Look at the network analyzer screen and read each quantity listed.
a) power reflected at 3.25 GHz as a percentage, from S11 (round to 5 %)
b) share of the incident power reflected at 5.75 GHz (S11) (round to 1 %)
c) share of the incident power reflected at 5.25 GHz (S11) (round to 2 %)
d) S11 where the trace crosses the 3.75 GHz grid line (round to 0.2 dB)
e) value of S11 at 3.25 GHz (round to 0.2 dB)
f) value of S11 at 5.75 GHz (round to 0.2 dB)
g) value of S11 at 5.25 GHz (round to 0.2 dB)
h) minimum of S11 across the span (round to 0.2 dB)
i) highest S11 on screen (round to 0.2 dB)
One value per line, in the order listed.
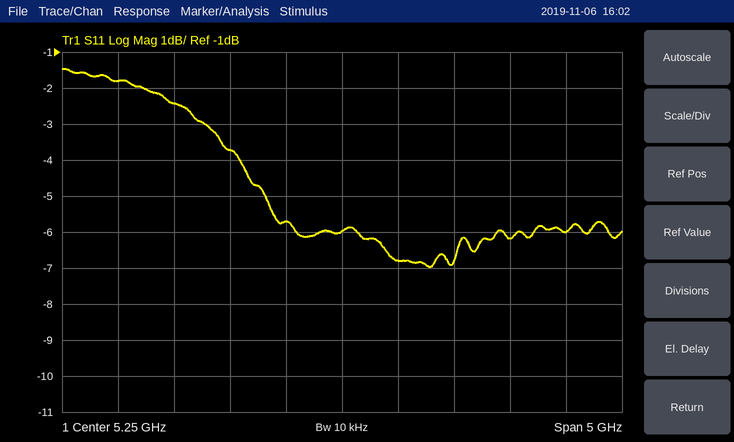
65 %
21 %
26 %
-2.4 dB
-1.8 dB
-6.8 dB
-6.0 dB
-7.0 dB
-1.4 dB
